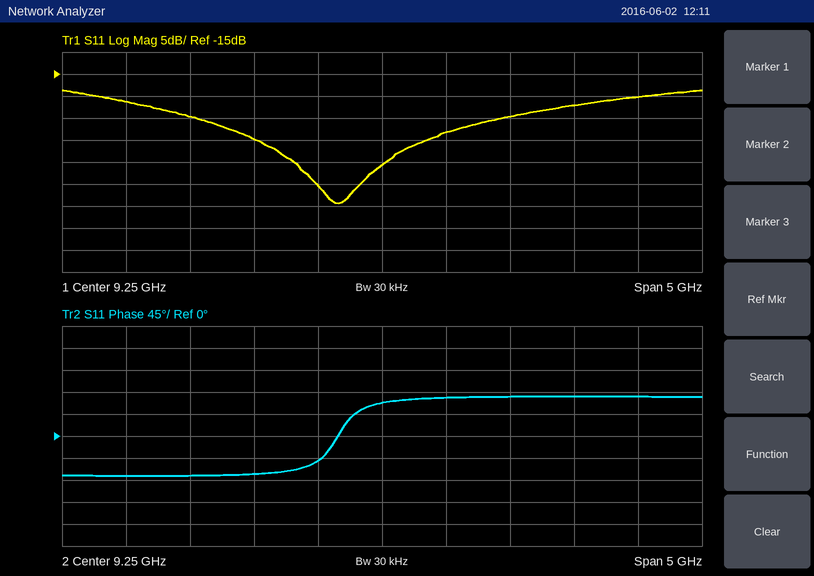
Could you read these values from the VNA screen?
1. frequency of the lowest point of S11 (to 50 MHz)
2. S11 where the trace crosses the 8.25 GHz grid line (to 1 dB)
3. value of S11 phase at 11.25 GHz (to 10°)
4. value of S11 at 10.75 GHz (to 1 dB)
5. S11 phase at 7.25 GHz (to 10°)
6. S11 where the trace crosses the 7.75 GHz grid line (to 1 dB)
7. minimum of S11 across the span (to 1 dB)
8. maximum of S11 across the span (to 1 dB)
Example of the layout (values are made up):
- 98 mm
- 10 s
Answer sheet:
- 8.90 GHz
- -30 dB
- 80°
- -22 dB
- -80°
- -25 dB
- -44 dB
- -19 dB
